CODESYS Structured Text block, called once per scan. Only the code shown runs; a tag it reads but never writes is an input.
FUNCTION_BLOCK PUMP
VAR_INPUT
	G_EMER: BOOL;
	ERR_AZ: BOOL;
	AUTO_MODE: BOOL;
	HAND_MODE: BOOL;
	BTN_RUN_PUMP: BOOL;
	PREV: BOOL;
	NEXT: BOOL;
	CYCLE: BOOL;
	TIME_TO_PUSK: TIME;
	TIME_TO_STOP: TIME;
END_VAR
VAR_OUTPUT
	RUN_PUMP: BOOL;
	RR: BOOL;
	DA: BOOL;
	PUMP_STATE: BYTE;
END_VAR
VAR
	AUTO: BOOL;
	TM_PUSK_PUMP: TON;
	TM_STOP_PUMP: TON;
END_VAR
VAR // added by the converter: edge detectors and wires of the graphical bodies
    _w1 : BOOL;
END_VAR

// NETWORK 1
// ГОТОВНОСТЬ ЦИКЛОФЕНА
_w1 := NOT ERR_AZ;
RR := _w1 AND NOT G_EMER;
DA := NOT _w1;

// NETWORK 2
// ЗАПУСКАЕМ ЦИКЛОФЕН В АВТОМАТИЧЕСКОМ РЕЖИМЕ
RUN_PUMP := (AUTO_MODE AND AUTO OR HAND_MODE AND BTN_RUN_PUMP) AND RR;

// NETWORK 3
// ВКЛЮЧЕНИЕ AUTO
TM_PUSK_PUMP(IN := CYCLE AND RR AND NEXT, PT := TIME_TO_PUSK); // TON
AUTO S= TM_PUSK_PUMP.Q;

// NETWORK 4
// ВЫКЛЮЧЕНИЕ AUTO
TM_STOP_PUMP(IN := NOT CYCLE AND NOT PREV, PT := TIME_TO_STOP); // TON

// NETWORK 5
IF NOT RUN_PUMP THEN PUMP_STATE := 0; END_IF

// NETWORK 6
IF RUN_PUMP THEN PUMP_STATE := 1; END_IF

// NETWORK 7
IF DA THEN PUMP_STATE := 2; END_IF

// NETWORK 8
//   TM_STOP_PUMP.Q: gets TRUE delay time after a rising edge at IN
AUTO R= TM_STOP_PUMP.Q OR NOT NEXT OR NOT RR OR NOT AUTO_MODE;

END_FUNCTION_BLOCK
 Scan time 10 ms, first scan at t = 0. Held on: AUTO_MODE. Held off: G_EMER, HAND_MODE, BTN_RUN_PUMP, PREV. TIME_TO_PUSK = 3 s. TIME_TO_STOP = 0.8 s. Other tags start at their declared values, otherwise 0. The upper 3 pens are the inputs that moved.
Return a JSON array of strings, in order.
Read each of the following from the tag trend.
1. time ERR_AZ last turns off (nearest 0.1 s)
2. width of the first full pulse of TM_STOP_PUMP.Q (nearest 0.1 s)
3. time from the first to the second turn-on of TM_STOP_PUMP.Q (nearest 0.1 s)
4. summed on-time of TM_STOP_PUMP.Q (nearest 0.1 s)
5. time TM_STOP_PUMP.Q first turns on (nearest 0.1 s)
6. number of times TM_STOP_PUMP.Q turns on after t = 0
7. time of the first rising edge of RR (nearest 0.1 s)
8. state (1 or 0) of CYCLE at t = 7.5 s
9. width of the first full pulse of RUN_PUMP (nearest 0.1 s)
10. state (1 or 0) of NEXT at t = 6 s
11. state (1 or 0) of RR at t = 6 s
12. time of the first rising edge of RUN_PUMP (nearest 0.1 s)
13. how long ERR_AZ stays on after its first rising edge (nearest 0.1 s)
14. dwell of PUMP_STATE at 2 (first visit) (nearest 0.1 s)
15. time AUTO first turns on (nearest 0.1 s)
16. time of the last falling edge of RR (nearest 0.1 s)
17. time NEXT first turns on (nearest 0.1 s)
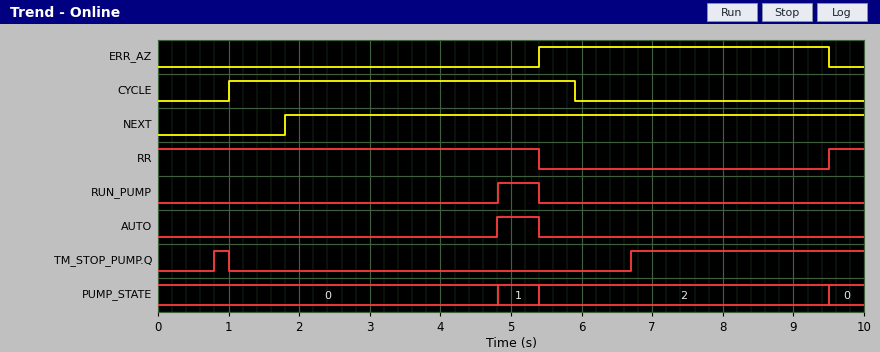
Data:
["9.5 s", "0.2 s", "5.9 s", "3.5 s", "0.8 s", "2", "9.5 s", "0", "0.6 s", "1", "0", "4.8 s", "4.1 s", "4.1 s", "4.8 s", "5.4 s", "1.8 s"]
